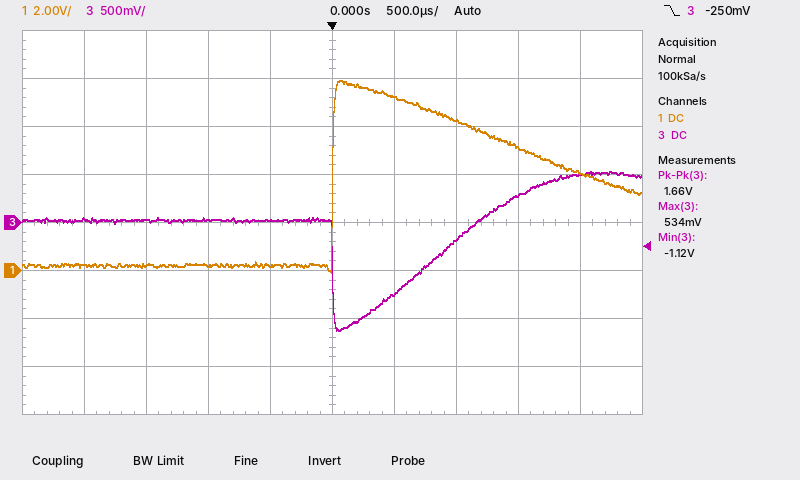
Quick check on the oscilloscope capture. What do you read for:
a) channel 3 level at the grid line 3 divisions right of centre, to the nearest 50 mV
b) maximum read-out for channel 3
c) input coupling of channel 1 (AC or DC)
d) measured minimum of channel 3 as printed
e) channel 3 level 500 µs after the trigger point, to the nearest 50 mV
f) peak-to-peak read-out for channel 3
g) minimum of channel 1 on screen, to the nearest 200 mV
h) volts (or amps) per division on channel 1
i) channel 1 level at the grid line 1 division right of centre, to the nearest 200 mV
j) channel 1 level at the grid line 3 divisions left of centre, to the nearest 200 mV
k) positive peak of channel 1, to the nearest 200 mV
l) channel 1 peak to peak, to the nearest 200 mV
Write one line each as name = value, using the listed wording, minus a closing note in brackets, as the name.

channel 3 level at the grid line 3 divisions right of centre, to the nearest 50 mV = 300 mV
maximum read-out for channel 3 = 534 mV
input coupling of channel 1 = DC
measured minimum of channel 3 as printed = -1.12 V
channel 3 level 500 µs after the trigger point, to the nearest 50 mV = -750 mV
peak-to-peak read-out for channel 3 = 1.66 V
minimum of channel 1 on screen, to the nearest 200 mV = 0.0 V
volts (or amps) per division on channel 1 = 2 V
channel 1 level at the grid line 1 division right of centre, to the nearest 200 mV = 7.2 V
channel 1 level at the grid line 3 divisions left of centre, to the nearest 200 mV = 200 mV
positive peak of channel 1, to the nearest 200 mV = 8.0 V
channel 1 peak to peak, to the nearest 200 mV = 8.0 V
